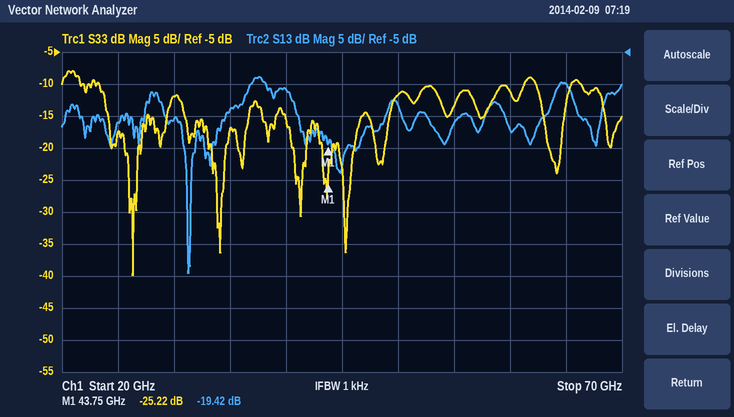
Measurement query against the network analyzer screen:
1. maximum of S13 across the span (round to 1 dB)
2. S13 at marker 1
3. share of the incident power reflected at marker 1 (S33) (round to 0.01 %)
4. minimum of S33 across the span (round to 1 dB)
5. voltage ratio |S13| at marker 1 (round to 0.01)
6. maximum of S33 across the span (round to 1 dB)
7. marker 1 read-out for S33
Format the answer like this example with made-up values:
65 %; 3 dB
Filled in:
-9 dB; -19.42 dB; 0.30 %; -40 dB; 0.11; -8 dB; -25.22 dB
